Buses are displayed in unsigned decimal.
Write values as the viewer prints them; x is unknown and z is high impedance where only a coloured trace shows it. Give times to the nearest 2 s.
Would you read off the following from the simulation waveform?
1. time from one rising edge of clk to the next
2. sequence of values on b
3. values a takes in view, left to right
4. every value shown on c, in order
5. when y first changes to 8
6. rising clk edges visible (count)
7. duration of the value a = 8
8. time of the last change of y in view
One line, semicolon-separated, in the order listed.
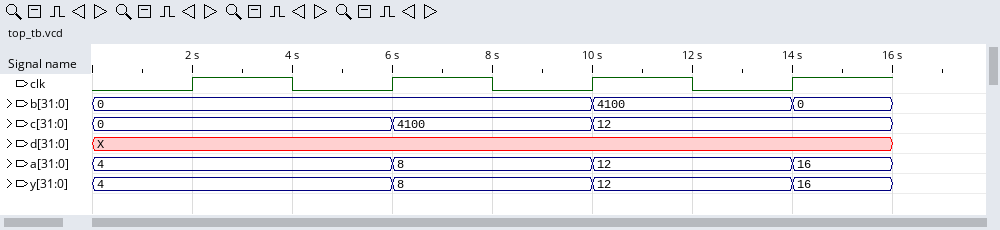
4 s; 0, 4100, 0; 4, 8, 12, 16; 0, 4100, 12; 6 s; 4; 4 s; 14 s
